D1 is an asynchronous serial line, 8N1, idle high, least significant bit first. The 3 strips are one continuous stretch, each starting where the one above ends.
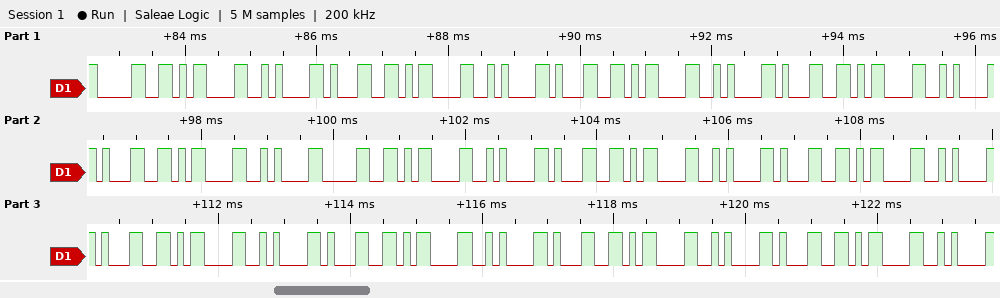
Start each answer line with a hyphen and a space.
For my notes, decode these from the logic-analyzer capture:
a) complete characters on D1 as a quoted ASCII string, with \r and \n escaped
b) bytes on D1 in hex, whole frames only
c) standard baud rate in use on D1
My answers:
- "0\r\n1\r\n1\r\n1\r\n1\r\n0\r\n1\r\n1\r\n1\r\n1\r\n1\r\n1\r\n"
- 30 0D 0A 31 0D 0A 31 0D 0A 31 0D 0A 31 0D 0A 30 0D 0A 31 0D 0A 31 0D 0A 31 0D 0A 31 0D 0A 31 0D 0A 31 0D 0A
- 9600 baud
